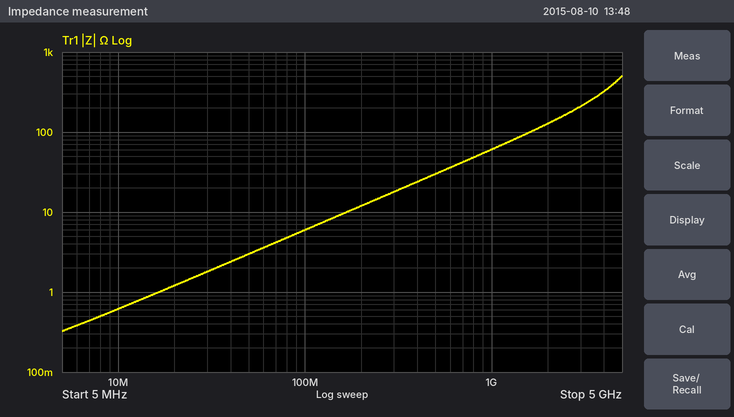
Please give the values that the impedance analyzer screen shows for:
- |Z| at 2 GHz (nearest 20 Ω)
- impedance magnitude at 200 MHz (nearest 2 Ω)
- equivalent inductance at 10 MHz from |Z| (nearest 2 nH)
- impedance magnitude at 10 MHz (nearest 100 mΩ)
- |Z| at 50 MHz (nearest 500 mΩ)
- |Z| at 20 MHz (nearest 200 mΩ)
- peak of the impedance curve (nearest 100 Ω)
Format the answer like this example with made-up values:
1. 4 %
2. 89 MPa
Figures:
1. 120 Ω
2. 12 Ω
3. 10 nH
4. 600 mΩ
5. 3.0 Ω
6. 1.2 Ω
7. 500 Ω
